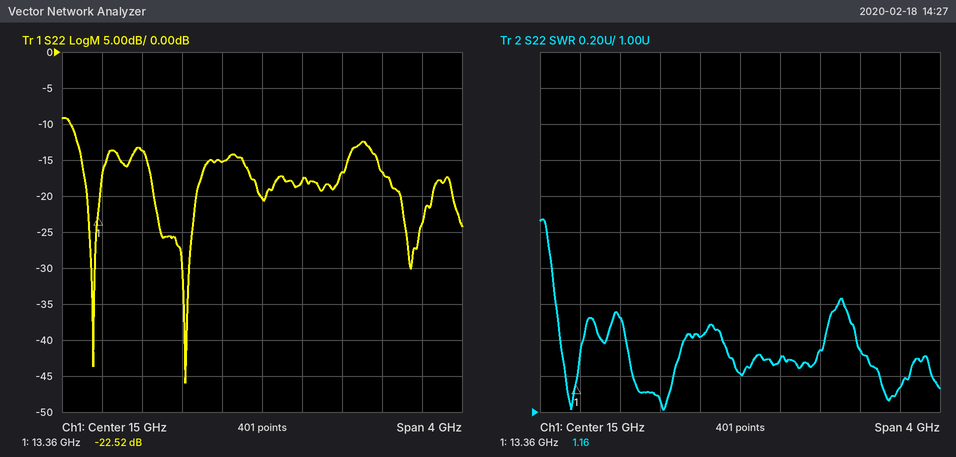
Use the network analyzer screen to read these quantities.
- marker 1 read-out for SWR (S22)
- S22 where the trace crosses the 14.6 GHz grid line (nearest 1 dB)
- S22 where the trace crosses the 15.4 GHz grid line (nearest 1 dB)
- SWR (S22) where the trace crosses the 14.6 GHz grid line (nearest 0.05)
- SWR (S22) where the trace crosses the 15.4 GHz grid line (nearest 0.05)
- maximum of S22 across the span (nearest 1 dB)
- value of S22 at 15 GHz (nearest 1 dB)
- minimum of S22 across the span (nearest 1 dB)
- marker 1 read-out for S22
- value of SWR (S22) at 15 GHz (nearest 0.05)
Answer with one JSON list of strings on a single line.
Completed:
["1.16", "-15 dB", "-18 dB", "1.40", "1.30", "-9 dB", "-20 dB", "-46 dB", "-22.52 dB", "1.20"]
